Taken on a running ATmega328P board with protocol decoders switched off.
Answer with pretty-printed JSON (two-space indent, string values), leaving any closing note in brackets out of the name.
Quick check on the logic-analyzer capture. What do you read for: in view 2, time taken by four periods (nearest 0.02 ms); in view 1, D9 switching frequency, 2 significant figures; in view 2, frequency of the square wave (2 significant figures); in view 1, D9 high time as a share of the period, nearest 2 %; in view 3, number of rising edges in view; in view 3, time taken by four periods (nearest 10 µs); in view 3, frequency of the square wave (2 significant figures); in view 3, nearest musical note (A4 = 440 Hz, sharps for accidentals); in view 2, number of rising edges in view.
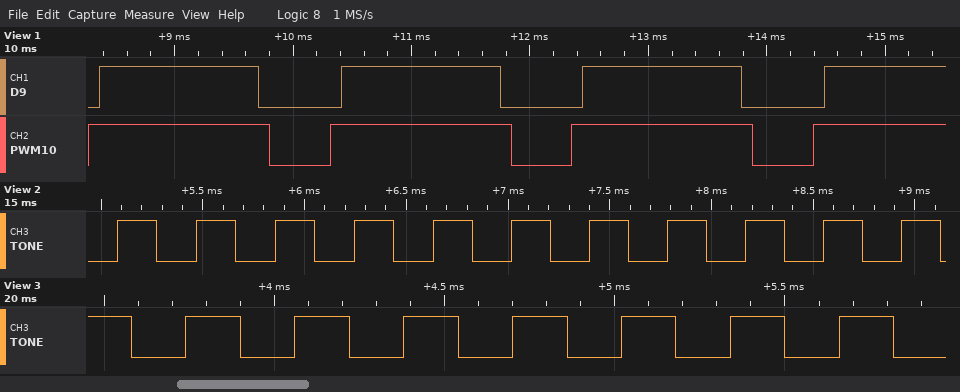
{
  "in view 2, time taken by four periods": "1.54 ms",
  "in view 1, D9 switching frequency, 2 significant figures": "490 Hz",
  "in view 2, frequency of the square wave": "2.6 kHz",
  "in view 1, D9 high time as a share of the period, nearest 2 %": "66 %",
  "in view 3, number of rising edges in view": "7",
  "in view 3, time taken by four periods": "1280 µs",
  "in view 3, frequency of the square wave": "3.1 kHz",
  "in view 3, nearest musical note": "G7",
  "in view 2, number of rising edges in view": "11"
}
